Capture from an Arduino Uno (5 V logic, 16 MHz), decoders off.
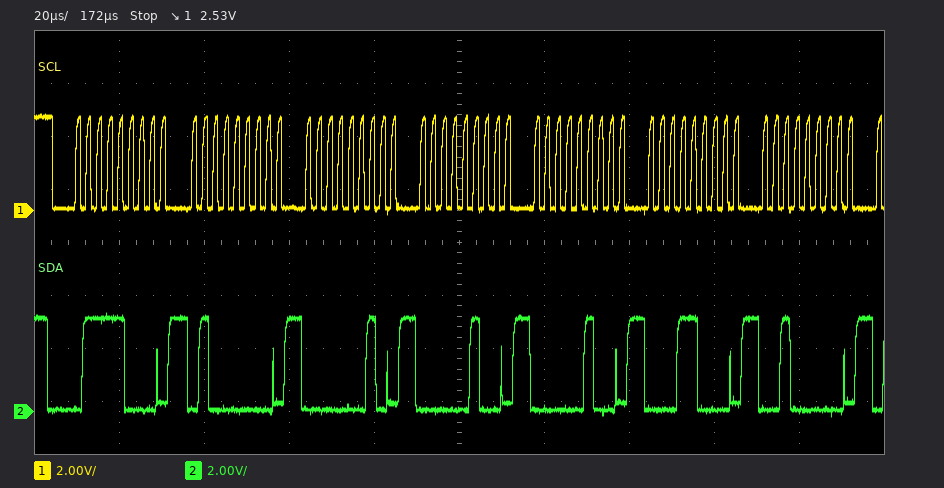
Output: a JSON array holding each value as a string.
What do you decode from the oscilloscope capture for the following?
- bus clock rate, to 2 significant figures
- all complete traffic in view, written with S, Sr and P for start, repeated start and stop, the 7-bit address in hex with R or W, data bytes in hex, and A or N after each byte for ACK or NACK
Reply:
["400 kHz", "S 3CW A 40 A 02 A 04 A 04 A 18 A 20 A"]
